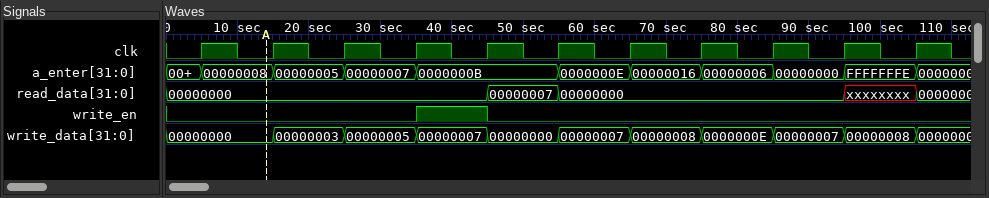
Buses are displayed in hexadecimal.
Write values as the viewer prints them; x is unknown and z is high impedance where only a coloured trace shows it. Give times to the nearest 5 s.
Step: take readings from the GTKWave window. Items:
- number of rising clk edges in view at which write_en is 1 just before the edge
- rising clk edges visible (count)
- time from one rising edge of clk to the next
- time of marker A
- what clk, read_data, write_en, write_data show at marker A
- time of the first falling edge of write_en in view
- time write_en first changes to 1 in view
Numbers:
1
11
10 s
15 s
clk=0, read_data=00000000, write_en=0, write_data=00000000
45 s
35 s
